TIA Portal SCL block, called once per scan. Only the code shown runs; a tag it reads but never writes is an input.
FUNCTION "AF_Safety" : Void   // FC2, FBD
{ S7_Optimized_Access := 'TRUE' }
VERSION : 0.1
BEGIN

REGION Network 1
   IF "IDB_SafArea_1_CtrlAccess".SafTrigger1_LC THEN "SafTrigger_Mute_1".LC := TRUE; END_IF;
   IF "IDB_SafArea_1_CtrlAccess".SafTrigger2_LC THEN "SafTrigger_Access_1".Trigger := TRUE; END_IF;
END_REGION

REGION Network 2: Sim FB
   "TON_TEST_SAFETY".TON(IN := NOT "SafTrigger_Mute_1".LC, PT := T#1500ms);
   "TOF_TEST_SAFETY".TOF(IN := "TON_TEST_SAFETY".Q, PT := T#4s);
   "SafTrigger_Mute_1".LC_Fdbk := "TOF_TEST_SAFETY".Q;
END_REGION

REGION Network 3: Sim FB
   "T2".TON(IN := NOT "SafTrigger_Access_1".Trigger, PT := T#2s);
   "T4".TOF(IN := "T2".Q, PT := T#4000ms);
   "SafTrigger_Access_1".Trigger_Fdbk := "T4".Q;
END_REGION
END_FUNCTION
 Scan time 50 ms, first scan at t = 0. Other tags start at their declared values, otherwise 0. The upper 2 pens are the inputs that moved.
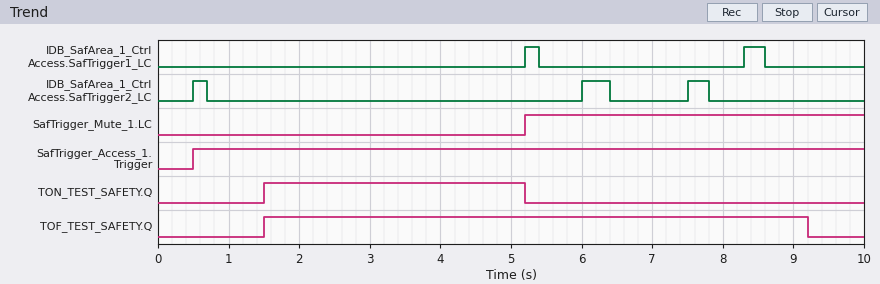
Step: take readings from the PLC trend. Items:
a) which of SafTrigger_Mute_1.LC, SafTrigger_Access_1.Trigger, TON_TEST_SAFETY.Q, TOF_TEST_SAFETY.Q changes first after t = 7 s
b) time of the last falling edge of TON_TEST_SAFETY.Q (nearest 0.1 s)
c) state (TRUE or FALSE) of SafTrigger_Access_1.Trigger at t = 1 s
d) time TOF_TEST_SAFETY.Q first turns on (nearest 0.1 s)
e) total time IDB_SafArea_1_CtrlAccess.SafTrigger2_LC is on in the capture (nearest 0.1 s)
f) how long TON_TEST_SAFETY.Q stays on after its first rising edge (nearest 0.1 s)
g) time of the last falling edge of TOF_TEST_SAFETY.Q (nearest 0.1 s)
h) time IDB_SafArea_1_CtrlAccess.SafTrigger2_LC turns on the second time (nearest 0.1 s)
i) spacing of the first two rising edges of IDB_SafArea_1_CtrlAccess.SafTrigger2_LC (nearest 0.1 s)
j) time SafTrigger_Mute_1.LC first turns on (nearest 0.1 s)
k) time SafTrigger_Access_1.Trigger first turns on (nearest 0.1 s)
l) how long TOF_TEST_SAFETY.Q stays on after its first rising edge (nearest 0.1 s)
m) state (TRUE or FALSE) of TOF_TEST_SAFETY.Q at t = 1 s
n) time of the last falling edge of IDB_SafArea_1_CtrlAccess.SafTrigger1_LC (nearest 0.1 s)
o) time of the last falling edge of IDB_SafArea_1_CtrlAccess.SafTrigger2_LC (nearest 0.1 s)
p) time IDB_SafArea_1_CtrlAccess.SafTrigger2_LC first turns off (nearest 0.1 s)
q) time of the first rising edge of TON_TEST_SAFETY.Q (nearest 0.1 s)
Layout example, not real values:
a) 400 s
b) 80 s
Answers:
a) TOF_TEST_SAFETY.Q
b) 5.2 s
c) TRUE
d) 1.5 s
e) 0.9 s
f) 3.7 s
g) 9.2 s
h) 6.0 s
i) 5.5 s
j) 5.2 s
k) 0.5 s
l) 7.7 s
m) FALSE
n) 8.6 s
o) 7.8 s
p) 0.7 s
q) 1.5 s
